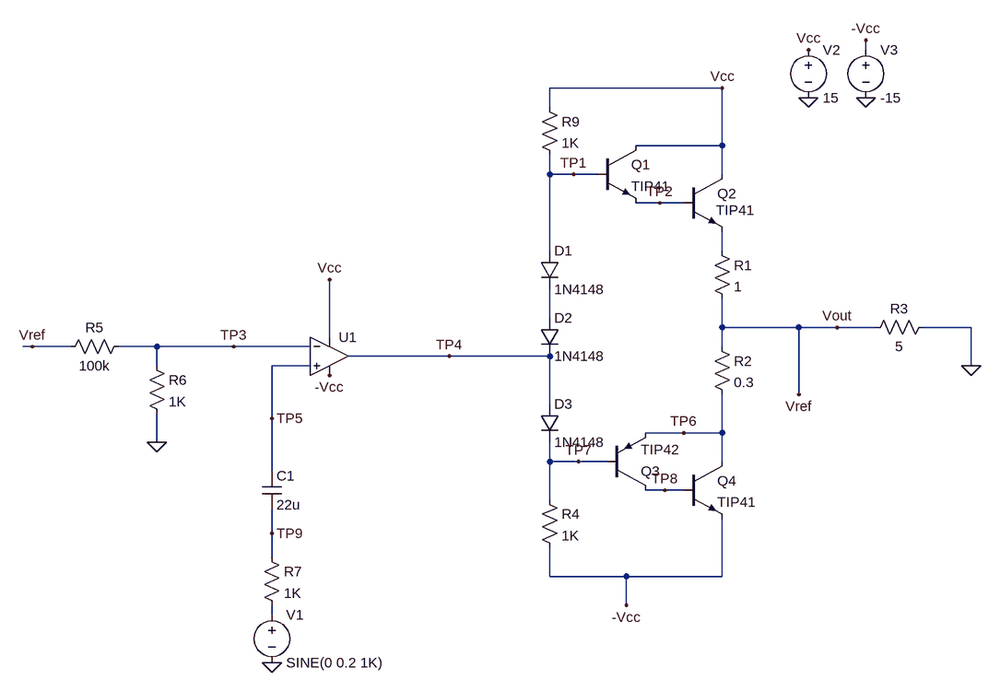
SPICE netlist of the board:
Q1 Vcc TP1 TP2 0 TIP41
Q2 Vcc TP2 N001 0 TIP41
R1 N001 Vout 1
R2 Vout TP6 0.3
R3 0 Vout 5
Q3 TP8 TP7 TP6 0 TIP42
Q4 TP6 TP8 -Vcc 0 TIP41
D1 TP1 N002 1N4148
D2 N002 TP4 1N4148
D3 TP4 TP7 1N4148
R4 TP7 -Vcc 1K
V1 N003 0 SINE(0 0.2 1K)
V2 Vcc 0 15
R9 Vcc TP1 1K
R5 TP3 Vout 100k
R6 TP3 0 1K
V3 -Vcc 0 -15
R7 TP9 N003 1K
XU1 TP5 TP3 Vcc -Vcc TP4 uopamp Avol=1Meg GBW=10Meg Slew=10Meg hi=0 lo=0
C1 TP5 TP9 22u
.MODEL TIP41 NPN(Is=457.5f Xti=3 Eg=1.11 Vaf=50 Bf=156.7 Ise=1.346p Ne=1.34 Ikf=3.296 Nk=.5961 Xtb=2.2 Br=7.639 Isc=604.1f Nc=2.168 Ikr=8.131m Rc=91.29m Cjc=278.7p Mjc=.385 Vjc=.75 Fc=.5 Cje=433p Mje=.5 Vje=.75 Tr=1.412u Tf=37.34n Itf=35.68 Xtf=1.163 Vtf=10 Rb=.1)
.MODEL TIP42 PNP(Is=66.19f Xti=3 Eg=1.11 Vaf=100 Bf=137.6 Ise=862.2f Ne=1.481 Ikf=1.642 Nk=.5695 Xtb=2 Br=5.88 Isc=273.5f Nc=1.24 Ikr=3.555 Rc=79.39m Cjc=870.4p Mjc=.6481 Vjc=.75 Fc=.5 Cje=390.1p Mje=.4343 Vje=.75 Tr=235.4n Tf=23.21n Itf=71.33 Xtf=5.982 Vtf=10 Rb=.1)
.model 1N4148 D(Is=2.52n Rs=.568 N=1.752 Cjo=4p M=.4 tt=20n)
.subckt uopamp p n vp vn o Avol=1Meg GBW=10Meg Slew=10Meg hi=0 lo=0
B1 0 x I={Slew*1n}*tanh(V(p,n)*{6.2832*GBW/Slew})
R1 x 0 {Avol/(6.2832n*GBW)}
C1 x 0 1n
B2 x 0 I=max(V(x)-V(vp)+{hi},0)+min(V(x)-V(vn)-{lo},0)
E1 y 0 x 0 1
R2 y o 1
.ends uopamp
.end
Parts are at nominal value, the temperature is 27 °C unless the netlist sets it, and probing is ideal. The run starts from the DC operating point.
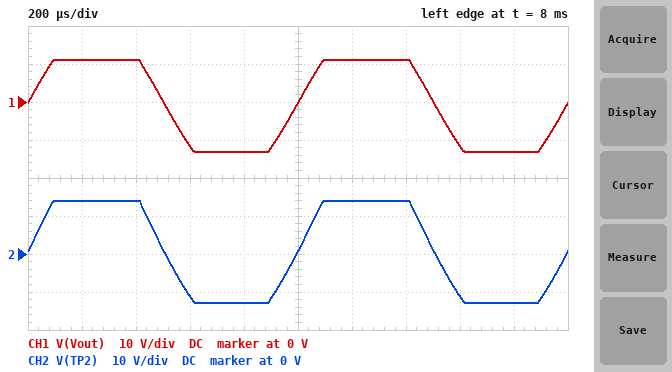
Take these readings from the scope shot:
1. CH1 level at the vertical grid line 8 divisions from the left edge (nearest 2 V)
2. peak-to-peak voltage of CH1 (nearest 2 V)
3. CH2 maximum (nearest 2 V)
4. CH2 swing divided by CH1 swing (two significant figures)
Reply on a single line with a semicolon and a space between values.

-12 V; 24 V; 14 V; 1.1
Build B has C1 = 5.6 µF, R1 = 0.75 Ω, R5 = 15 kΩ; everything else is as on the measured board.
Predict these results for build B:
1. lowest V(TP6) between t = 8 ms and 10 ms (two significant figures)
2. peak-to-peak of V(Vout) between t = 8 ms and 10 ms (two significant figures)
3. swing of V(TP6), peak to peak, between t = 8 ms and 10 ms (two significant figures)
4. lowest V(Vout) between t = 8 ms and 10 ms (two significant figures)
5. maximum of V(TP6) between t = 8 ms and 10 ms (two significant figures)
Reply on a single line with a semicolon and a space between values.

-3.4 V; 6.4 V; 6.6 V; -3.2 V; 3.2 V
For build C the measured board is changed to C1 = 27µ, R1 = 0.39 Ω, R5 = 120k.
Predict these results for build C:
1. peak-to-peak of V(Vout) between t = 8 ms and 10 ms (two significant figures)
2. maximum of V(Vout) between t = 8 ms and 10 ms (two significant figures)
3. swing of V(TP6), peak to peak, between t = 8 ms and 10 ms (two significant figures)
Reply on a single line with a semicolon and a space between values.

25 V; 12 V; 26 V
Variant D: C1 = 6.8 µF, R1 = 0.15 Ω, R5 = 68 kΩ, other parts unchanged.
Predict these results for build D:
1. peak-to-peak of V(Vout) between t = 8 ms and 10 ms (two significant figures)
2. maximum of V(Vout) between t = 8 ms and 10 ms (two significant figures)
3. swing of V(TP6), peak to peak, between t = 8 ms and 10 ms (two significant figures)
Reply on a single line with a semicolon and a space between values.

26 V; 13 V; 27 V
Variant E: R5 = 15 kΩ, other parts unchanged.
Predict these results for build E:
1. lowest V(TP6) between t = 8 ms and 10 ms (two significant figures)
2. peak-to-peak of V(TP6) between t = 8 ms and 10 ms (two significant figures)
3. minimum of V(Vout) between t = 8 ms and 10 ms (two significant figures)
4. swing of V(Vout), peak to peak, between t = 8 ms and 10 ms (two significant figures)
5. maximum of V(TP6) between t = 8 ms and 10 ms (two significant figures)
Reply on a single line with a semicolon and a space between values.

-3.4 V; 6.6 V; -3.2 V; 6.4 V; 3.2 V
